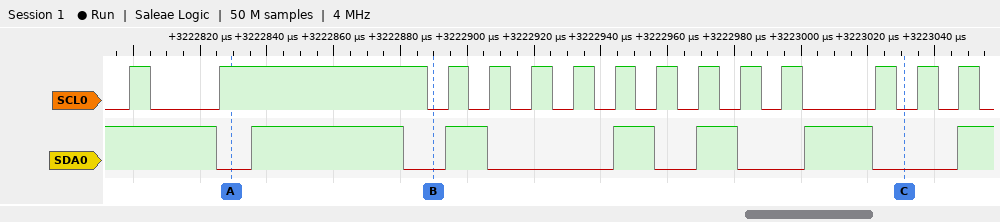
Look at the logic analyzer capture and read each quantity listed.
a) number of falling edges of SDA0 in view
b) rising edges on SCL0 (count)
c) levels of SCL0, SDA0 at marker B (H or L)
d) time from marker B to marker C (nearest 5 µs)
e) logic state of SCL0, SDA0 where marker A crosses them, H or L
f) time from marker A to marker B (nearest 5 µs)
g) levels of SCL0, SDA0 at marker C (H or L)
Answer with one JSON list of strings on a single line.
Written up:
["6", "14", "SCL0=L, SDA0=L", "140 µs", "SCL0=H, SDA0=L", "60 µs", "SCL0=L, SDA0=L"]
